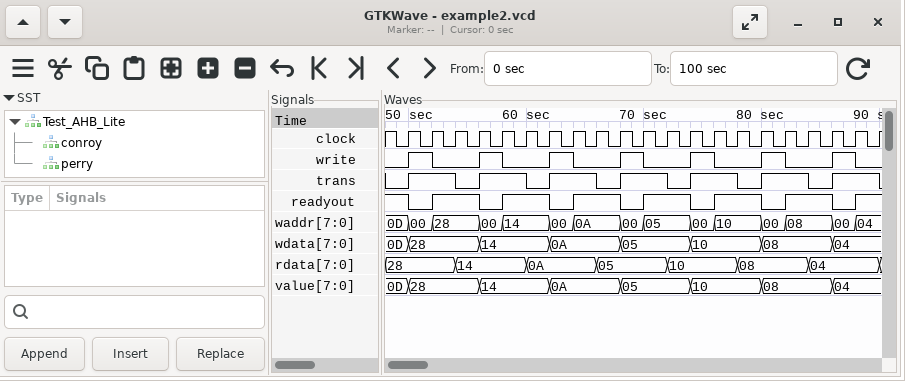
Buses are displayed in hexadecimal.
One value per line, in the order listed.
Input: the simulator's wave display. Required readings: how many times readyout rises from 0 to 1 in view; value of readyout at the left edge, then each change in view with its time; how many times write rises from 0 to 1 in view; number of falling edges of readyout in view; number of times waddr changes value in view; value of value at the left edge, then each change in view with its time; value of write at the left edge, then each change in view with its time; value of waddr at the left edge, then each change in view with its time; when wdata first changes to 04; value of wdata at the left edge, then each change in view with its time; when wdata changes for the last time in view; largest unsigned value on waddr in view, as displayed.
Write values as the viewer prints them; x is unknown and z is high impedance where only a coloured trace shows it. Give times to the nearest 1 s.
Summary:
7
1, 0 at 50 s, 1 at 52 s, 0 at 56 s, 1 at 58 s, 0 at 62 s, 1 at 64 s, 0 at 68 s, 1 at 70 s, 0 at 74 s, 1 at 76 s, 0 at 80 s, 1 at 82 s, 0 at 86 s, 1 at 88 s
7
7
14
0D, 28 at 50 s, 14 at 56 s, 0A at 62 s, 05 at 68 s, 10 at 74 s, 08 at 80 s, 04 at 86 s
0, 1 at 50 s, 0 at 52 s, 1 at 56 s, 0 at 58 s, 1 at 62 s, 0 at 64 s, 1 at 68 s, 0 at 70 s, 1 at 74 s, 0 at 76 s, 1 at 80 s, 0 at 82 s, 1 at 86 s, 0 at 88 s
0D, 00 at 50 s, 28 at 52 s, 00 at 56 s, 14 at 58 s, 00 at 62 s, 0A at 64 s, 00 at 68 s, 05 at 70 s, 00 at 74 s, 10 at 76 s, 00 at 80 s, 08 at 82 s, 00 at 86 s, 04 at 88 s
86 s
0D, 28 at 50 s, 14 at 56 s, 0A at 62 s, 05 at 68 s, 10 at 74 s, 08 at 80 s, 04 at 86 s
86 s
28
